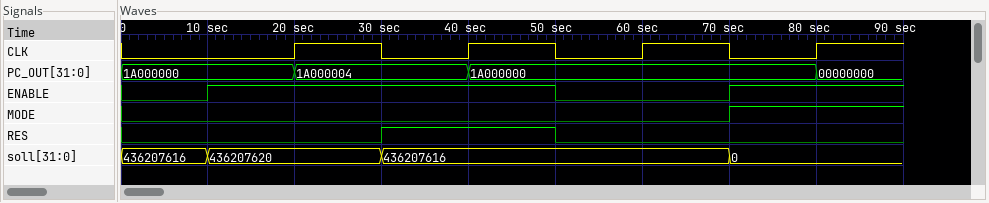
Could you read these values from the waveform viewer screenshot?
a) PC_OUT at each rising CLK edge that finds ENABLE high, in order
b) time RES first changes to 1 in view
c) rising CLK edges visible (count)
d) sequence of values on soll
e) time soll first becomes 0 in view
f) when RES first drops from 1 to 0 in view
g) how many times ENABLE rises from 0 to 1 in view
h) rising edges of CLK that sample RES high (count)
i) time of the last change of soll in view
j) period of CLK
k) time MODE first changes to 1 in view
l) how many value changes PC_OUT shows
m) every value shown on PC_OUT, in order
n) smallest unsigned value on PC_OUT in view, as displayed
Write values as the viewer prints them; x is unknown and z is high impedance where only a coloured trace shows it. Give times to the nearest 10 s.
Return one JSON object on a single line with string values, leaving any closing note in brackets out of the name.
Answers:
{"PC_OUT at each rising CLK edge that finds ENABLE high, in order": "1A000000, 1A000004, 1A000000", "time RES first changes to 1 in view": "30 s", "rising CLK edges visible": "4", "sequence of values on soll": "436207616, 436207620, 436207616, 0", "time soll first becomes 0 in view": "70 s", "when RES first drops from 1 to 0 in view": "50 s", "how many times ENABLE rises from 0 to 1 in view": "2", "rising edges of CLK that sample RES high": "1", "time of the last change of soll in view": "70 s", "period of CLK": "20 s", "time MODE first changes to 1 in view": "70 s", "how many value changes PC_OUT shows": "3", "every value shown on PC_OUT, in order": "1A000000, 1A000004, 1A000000, 00000000", "smallest unsigned value on PC_OUT in view, as displayed": "00000000"}
